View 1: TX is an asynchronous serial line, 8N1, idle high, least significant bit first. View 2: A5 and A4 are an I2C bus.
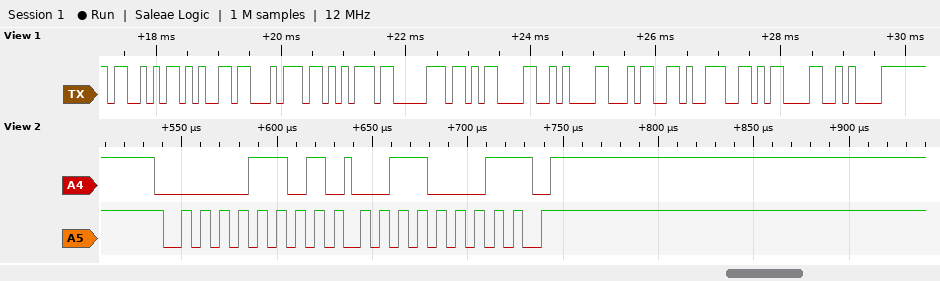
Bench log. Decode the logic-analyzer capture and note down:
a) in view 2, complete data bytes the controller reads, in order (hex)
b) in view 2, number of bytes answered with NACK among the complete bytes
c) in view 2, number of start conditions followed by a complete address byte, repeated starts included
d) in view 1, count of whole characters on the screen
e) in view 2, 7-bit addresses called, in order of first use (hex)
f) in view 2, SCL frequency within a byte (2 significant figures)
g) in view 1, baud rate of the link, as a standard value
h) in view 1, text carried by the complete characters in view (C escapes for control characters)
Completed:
31
1
1
11
0x06
100 kHz
9600 baud
"Setup\r\n49\r\n"
